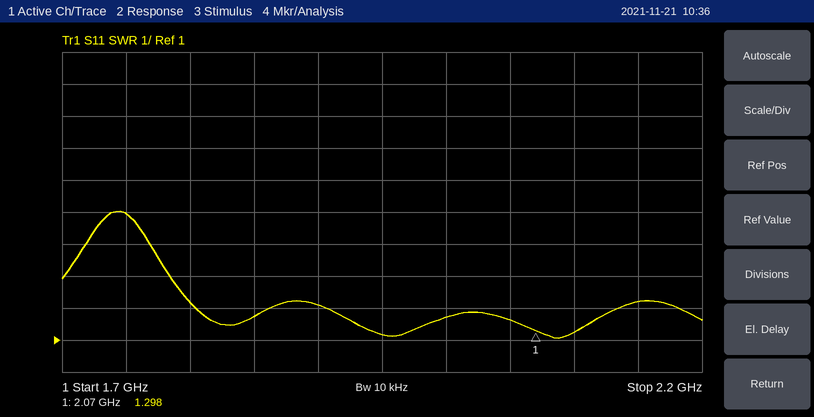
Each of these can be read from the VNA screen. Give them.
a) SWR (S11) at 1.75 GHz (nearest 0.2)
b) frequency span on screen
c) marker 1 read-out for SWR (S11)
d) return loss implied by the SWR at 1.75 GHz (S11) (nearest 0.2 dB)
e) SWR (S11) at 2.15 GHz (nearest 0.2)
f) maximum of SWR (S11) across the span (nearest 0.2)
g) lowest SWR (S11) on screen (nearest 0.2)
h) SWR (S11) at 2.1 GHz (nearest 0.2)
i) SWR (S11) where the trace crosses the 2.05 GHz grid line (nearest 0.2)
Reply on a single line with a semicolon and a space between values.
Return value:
5.0; 500 MHz; 1.298; 3.6 dB; 2.2; 5.0; 1.0; 1.2; 1.6
